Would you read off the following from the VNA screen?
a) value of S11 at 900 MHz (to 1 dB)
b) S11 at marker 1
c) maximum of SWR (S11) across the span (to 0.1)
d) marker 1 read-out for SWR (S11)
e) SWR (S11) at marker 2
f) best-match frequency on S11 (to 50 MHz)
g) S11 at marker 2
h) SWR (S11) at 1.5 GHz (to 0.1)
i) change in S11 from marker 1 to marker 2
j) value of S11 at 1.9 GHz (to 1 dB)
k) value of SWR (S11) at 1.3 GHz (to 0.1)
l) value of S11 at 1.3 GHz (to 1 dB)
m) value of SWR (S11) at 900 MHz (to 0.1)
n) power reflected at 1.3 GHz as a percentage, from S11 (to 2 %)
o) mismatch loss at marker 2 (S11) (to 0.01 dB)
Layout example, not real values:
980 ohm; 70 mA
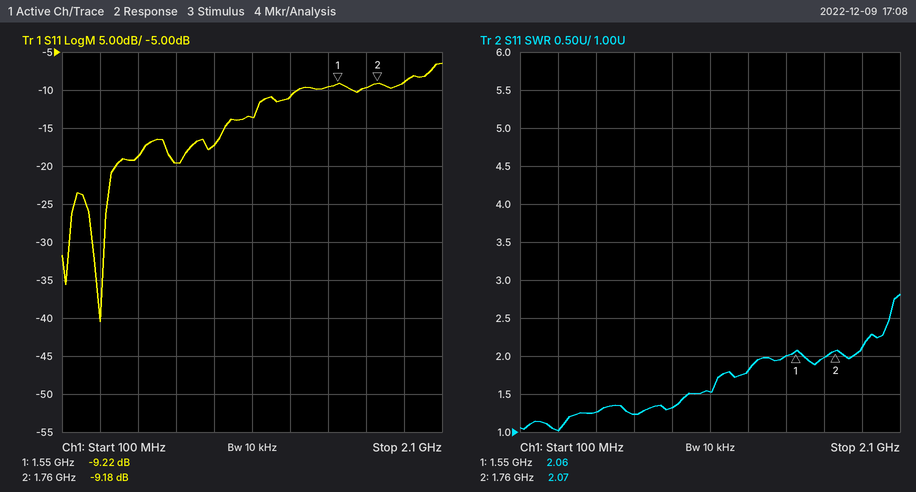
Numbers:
-17 dB; -9.22 dB; 2.8; 2.06; 2.07; 300 MHz; -9.18 dB; 2.0; 0.04 dB; -9 dB; 1.8; -11 dB; 1.3; 8 %; 0.56 dB
